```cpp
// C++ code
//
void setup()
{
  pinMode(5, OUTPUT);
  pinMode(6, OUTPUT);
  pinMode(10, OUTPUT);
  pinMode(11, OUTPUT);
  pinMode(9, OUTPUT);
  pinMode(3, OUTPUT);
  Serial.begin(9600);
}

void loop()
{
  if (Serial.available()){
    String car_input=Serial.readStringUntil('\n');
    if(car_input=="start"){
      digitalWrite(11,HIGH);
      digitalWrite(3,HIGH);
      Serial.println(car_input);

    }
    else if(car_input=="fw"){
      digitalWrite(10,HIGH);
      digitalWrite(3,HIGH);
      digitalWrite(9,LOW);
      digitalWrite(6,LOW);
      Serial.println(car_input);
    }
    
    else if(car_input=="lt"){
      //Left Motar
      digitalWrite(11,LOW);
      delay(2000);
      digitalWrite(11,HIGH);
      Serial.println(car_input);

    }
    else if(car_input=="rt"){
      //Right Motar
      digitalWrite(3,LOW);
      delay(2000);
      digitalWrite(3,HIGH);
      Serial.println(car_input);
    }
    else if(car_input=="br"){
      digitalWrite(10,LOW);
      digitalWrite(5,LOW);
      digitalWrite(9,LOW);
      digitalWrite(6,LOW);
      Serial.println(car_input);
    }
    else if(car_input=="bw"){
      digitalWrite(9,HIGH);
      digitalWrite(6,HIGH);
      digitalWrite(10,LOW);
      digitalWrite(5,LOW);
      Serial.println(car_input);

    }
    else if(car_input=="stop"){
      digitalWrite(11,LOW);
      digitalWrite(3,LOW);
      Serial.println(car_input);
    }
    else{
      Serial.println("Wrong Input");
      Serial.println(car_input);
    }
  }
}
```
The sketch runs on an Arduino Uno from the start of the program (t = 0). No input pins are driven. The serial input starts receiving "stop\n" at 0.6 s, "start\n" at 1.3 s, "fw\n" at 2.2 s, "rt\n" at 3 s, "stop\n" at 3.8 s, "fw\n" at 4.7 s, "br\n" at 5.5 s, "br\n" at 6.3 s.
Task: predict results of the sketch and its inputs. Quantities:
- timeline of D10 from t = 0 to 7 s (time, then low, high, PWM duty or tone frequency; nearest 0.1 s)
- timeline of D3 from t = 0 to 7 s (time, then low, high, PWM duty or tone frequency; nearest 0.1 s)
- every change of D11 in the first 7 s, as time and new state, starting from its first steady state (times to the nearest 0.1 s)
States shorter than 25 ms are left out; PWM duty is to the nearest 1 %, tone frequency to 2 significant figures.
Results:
0 s low; 2.2 s high; 5.5 s low
0 s low; 1.3 s high; 3 s low; 5 s high
0 s low; 1.3 s high; 5 s low
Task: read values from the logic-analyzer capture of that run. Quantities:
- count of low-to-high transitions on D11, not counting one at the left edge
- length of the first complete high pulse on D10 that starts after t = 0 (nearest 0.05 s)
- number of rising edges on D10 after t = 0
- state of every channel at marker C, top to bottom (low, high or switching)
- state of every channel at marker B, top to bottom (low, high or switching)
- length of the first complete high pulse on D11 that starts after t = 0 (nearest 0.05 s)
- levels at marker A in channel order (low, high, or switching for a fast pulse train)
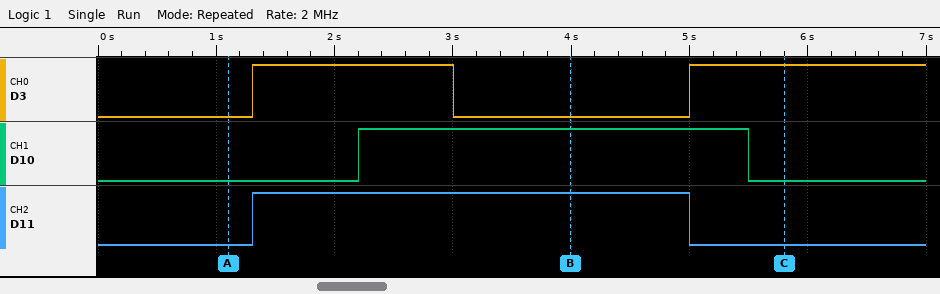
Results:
1
3.30 s
1
D3 high, D10 low, D11 low
D3 low, D10 high, D11 high
3.70 s
D3 low, D10 low, D11 low
